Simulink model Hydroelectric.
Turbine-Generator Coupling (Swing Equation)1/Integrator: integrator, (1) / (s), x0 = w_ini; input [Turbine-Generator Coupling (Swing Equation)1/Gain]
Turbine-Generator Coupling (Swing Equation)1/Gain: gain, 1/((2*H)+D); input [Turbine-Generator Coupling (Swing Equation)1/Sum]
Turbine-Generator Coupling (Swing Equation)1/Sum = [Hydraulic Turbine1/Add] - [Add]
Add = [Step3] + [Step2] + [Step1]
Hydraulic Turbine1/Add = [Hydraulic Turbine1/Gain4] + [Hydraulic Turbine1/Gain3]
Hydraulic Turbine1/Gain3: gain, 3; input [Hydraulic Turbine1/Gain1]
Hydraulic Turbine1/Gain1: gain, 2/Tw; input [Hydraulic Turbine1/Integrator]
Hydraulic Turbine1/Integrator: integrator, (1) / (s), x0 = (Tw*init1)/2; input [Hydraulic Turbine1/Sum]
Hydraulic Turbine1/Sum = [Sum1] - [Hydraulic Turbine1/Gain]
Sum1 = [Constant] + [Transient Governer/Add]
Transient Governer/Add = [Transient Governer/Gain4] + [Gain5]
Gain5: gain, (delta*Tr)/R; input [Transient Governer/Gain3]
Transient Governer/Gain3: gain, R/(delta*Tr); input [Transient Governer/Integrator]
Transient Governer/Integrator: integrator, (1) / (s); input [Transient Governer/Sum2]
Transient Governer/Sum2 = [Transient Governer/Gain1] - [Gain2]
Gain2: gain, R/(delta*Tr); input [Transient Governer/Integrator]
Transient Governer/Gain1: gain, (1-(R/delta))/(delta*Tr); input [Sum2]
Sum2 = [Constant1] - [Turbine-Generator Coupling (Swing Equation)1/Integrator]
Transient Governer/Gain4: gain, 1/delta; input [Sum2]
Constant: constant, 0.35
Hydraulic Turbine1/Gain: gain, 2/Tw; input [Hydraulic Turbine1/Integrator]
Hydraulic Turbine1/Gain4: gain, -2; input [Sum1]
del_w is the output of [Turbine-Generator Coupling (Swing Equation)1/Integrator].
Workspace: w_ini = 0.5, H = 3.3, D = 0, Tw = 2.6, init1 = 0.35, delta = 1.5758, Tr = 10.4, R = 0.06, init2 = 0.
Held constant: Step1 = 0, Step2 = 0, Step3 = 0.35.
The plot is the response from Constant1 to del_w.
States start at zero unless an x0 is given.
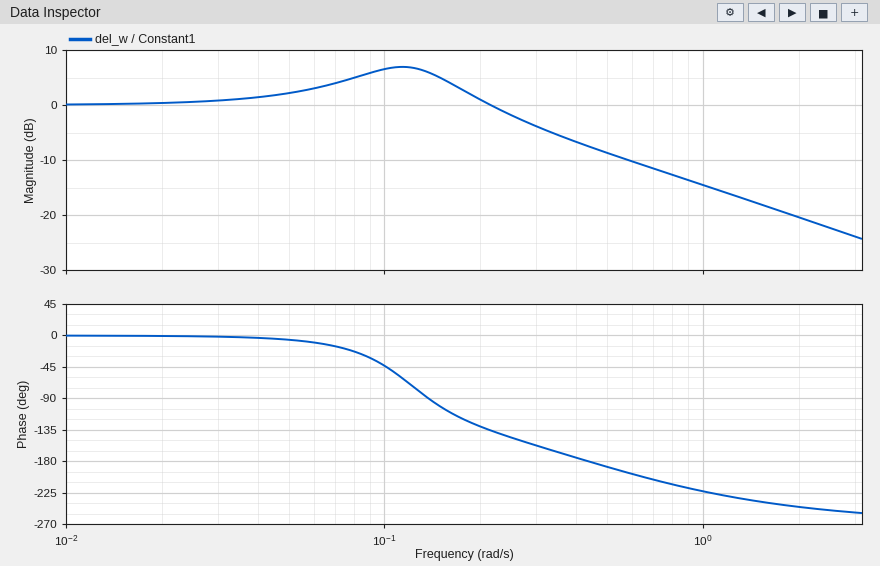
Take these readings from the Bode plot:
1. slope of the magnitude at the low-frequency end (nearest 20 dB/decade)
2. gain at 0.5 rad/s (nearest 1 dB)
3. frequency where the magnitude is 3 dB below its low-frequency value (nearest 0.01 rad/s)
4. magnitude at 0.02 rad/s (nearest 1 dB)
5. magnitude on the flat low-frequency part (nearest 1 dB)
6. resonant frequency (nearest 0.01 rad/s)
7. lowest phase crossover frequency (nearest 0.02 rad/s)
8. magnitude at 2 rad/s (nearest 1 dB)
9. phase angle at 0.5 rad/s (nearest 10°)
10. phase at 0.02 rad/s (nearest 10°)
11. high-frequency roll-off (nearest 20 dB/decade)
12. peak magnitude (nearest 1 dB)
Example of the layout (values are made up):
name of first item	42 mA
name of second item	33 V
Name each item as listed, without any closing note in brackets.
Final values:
slope of the magnitude at the low-frequency end	0 dB/decade
gain at 0.5 rad/s	-9 dB
frequency where the magnitude is 3 dB below its low-frequency value	0.27 rad/s
magnitude at 0.02 rad/s	0 dB
magnitude on the flat low-frequency part	0 dB
resonant frequency	0.11 rad/s
lowest phase crossover frequency	0.44 rad/s
magnitude at 2 rad/s	-20 dB
phase angle at 0.5 rad/s	-190°
phase at 0.02 rad/s	0°
high-frequency roll-off	-20 dB/decade
peak magnitude	7 dB
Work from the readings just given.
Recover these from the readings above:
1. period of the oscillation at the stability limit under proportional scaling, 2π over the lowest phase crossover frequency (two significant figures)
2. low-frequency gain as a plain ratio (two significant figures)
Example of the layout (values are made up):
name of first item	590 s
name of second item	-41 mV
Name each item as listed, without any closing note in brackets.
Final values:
period of the oscillation at the stability limit under proportional scaling, 2π over the lowest phase crossover frequency	14 s
low-frequency gain as a plain ratio	1.0
